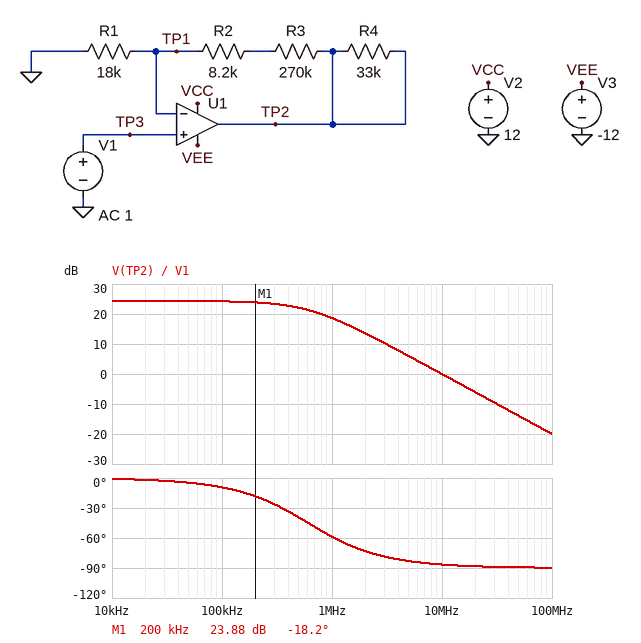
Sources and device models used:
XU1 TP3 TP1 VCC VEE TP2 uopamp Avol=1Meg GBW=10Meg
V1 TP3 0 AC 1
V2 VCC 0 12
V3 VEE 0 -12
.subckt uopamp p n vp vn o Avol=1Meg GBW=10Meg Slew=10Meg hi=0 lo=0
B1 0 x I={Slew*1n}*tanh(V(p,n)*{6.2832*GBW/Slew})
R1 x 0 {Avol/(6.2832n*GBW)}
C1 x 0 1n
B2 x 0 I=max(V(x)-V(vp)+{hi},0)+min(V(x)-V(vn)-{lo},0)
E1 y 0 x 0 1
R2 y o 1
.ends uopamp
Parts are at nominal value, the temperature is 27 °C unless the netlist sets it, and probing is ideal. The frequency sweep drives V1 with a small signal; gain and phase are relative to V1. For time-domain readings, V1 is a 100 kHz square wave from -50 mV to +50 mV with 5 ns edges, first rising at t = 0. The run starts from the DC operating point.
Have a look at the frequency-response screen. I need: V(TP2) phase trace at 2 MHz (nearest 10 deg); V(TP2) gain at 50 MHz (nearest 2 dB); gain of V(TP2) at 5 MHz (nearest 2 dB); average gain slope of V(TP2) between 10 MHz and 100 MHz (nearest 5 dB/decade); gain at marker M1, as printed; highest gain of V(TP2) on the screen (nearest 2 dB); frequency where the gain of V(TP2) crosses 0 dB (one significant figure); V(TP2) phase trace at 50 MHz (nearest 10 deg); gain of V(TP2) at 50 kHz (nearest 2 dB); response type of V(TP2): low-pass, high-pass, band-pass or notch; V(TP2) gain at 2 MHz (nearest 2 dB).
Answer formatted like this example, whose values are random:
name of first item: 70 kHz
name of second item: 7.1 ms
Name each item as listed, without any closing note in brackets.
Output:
V(TP2) phase trace at 2 MHz: -70 deg
V(TP2) gain at 50 MHz: -14 dB
gain of V(TP2) at 5 MHz: 6 dB
average gain slope of V(TP2) between 10 MHz and 100 MHz: -20 dB/decade
gain at marker M1, as printed: 23.88 dB
highest gain of V(TP2) on the screen: 24 dB
frequency where the gain of V(TP2) crosses 0 dB: 10 MHz
V(TP2) phase trace at 50 MHz: -90 deg
gain of V(TP2) at 50 kHz: 24 dB
response type of V(TP2): low-pass, high-pass, band-pass or notch: low-pass
V(TP2) gain at 2 MHz: 14 dB
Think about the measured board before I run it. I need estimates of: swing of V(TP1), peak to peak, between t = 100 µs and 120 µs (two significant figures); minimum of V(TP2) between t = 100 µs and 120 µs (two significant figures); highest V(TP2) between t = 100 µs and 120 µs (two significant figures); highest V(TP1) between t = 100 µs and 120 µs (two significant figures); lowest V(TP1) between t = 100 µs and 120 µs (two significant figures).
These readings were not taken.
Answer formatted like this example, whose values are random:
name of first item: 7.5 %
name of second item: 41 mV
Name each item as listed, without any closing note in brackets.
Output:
swing of V(TP1), peak to peak, between t = 100 µs and 120 µs: 100 mV
minimum of V(TP2) between t = 100 µs and 120 µs: -820 mV
highest V(TP2) between t = 100 µs and 120 µs: 820 mV
highest V(TP1) between t = 100 µs and 120 µs: 50 mV
lowest V(TP1) between t = 100 µs and 120 µs: -50 mV
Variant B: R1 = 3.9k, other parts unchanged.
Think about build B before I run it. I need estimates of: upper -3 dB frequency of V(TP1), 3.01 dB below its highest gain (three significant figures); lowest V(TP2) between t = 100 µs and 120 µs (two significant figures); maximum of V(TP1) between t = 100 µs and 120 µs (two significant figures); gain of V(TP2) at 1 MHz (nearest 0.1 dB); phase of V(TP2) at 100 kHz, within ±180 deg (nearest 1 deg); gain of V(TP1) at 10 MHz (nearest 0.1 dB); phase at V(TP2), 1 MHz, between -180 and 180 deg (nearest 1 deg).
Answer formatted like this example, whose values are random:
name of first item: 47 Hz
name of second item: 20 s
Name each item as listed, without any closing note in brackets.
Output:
upper -3 dB frequency of V(TP1), 3.01 dB below its highest gain: 138 kHz
lowest V(TP2) between t = 100 µs and 120 µs: -3.5 V
maximum of V(TP1) between t = 100 µs and 120 µs: 49 mV
gain of V(TP2) at 1 MHz: 19.9 dB
phase of V(TP2) at 100 kHz, within ±180 deg: -36 deg
gain of V(TP1) at 10 MHz: -37.2 dB
phase at V(TP2), 1 MHz, between -180 and 180 deg: -82 deg
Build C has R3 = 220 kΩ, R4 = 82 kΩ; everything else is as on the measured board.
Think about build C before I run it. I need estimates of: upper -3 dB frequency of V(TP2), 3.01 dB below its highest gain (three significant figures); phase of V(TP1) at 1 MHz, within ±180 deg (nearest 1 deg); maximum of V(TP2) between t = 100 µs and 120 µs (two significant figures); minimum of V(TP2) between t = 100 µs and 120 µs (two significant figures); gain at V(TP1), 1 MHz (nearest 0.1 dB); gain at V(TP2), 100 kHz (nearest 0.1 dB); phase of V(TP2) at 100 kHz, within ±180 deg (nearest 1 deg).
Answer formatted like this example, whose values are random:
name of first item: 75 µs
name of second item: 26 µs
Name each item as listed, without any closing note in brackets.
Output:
upper -3 dB frequency of V(TP2), 3.01 dB below its highest gain: 731 kHz
phase of V(TP1) at 1 MHz, within ±180 deg: -54 deg
maximum of V(TP2) between t = 100 µs and 120 µs: 680 mV
minimum of V(TP2) between t = 100 µs and 120 µs: -680 mV
gain at V(TP1), 1 MHz: -4.6 dB
gain at V(TP2), 100 kHz: 22.6 dB
phase of V(TP2) at 100 kHz, within ±180 deg: -8 deg
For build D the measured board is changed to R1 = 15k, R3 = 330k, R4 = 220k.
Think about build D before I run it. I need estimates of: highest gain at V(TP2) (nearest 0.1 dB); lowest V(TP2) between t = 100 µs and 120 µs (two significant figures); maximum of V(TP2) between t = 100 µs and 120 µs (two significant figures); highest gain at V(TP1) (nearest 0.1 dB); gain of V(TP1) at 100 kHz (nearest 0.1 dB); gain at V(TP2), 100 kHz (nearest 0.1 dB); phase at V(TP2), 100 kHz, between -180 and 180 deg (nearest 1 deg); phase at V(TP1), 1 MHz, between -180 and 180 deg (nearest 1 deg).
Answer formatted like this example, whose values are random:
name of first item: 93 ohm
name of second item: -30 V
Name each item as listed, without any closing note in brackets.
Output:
highest gain at V(TP2): 27.4 dB
lowest V(TP2) between t = 100 µs and 120 µs: -1.2 V
maximum of V(TP2) between t = 100 µs and 120 µs: 1.2 V
highest gain at V(TP1): 0 dB
gain of V(TP1) at 100 kHz: -0.2 dB
gain at V(TP2), 100 kHz: 27.2 dB
phase at V(TP2), 100 kHz, between -180 and 180 deg: -13 deg
phase at V(TP1), 1 MHz, between -180 and 180 deg: -67 deg
